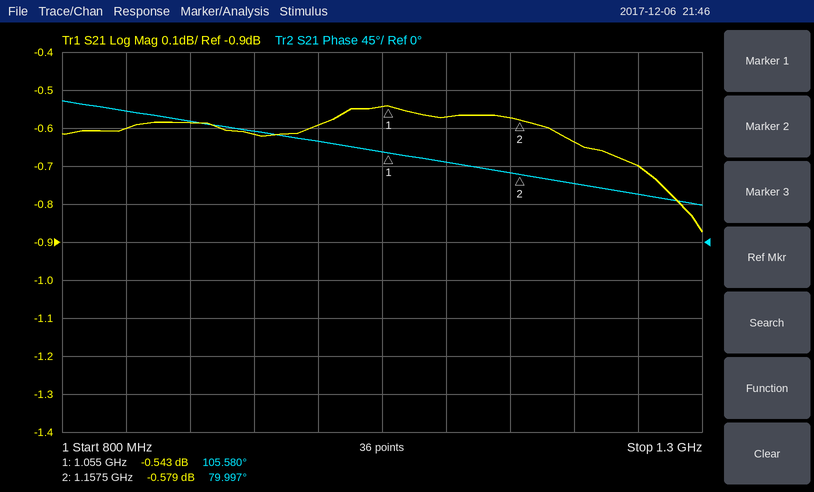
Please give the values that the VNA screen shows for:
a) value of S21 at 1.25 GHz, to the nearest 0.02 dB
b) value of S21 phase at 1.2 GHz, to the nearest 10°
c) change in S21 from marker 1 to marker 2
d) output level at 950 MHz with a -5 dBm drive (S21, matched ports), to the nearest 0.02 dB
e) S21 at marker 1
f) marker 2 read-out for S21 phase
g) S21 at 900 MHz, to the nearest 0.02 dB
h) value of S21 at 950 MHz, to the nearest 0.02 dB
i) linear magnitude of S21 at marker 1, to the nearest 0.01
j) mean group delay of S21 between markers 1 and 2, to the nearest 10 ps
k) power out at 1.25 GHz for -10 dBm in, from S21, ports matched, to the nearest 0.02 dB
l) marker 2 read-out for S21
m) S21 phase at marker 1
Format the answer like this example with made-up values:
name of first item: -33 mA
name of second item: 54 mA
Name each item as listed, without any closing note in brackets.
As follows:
value of S21 at 1.25 GHz, to the nearest 0.02 dB: -0.70 dB
value of S21 phase at 1.2 GHz, to the nearest 10°: 70°
change in S21 from marker 1 to marker 2: -0.036 dB
output level at 950 MHz with a -5 dBm drive (S21, matched ports), to the nearest 0.02 dB: -5.62 dBm
S21 at marker 1: -0.543 dB
marker 2 read-out for S21 phase: 79.997°
S21 at 900 MHz, to the nearest 0.02 dB: -0.58 dB
value of S21 at 950 MHz, to the nearest 0.02 dB: -0.62 dB
linear magnitude of S21 at marker 1, to the nearest 0.01: 0.94
mean group delay of S21 between markers 1 and 2, to the nearest 10 ps: 690 ps
power out at 1.25 GHz for -10 dBm in, from S21, ports matched, to the nearest 0.02 dB: -10.70 dBm
marker 2 read-out for S21: -0.579 dB
S21 phase at marker 1: 105.580°
